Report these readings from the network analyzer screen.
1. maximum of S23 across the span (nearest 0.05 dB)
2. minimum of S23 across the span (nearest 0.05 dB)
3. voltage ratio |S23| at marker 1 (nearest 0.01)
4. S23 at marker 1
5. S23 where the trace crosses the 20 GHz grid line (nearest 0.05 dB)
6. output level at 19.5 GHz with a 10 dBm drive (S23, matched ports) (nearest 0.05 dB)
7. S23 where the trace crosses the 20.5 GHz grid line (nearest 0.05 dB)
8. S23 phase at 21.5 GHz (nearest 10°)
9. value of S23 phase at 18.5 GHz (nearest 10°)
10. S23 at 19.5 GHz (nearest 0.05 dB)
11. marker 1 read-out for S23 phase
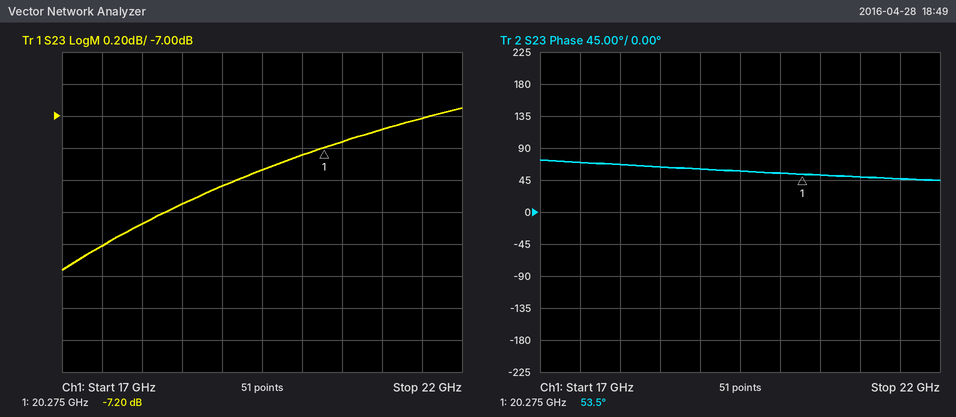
-6.95 dB
-7.95 dB
0.44
-7.20 dB
-7.25 dB
2.65 dBm
-7.15 dB
50°
60°
-7.35 dB
53.5°
